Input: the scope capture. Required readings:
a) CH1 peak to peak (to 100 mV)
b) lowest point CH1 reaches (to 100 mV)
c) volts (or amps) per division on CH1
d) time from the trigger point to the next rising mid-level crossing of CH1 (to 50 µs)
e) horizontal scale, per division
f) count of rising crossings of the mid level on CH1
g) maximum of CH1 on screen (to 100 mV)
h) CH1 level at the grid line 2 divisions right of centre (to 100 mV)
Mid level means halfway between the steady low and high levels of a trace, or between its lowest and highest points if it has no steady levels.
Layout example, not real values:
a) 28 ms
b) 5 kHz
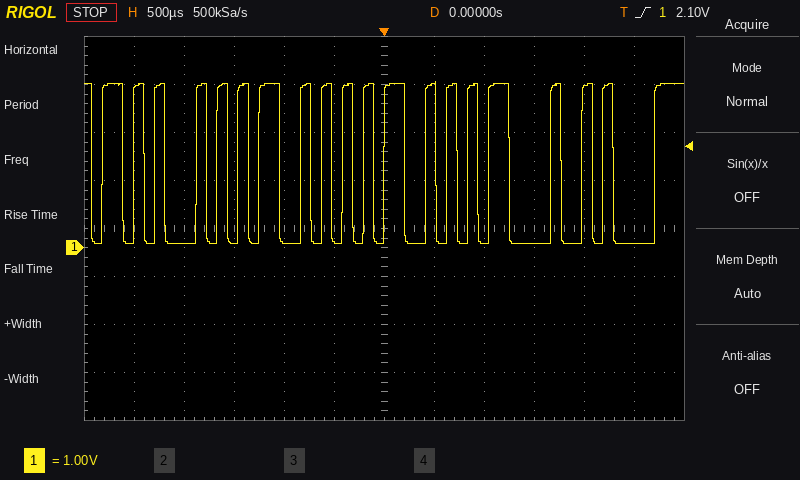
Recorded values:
a) 3.4 V
b) 100 mV
c) 1 V
d) 400 µs
e) 500 µs
f) 20
g) 3.5 V
h) 100 mV
